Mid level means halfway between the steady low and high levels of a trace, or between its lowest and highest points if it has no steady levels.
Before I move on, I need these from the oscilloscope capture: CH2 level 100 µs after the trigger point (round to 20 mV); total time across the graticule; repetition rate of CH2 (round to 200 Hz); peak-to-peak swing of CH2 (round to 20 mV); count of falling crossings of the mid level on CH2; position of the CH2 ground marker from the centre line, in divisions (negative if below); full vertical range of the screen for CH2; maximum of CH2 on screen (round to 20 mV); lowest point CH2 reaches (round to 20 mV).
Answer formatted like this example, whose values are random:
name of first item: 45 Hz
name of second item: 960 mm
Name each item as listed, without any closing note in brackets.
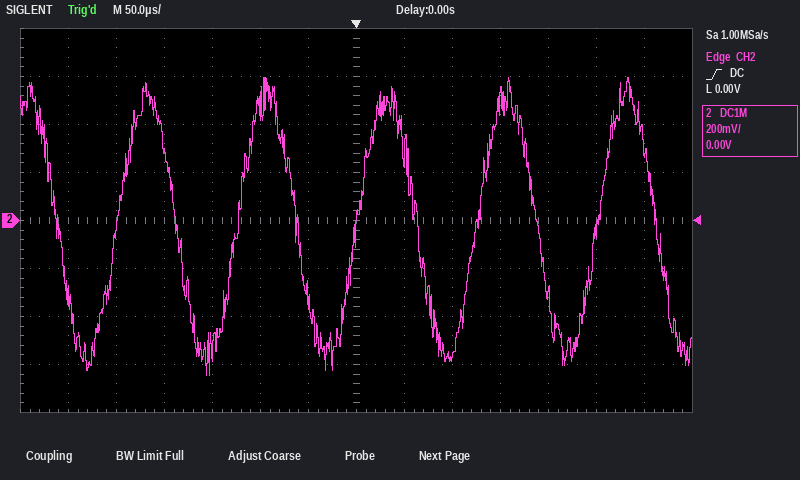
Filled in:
CH2 level 100 µs after the trigger point: -560 mV
total time across the graticule: 700 µs
repetition rate of CH2: 8.0 kHz
peak-to-peak swing of CH2: 1.24 V
count of falling crossings of the mid level on CH2: 6
position of the CH2 ground marker from the centre line, in divisions: 0.0 div
full vertical range of the screen for CH2: 1.6 V
maximum of CH2 on screen: 600 mV
lowest point CH2 reaches: -640 mV
